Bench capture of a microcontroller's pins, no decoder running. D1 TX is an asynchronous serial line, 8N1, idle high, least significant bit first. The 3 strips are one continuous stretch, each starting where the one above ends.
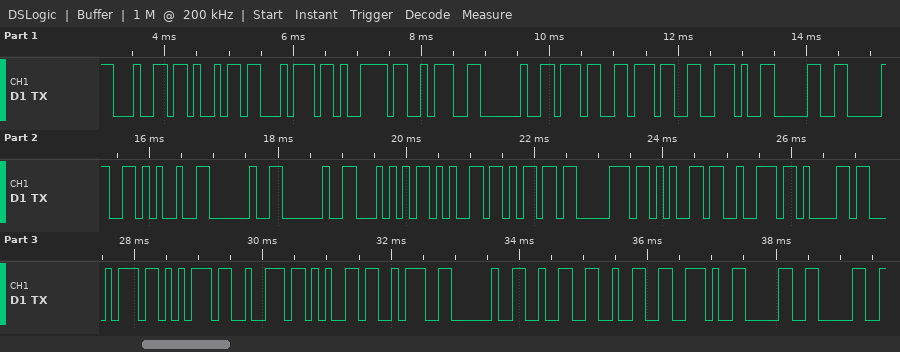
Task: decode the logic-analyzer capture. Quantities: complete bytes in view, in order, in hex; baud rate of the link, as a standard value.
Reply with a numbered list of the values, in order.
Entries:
1. 64 69 74 79 3A 20 37 37 2E 30 30 25 20 20 54 65 6D 70 65 72 61 74 75 72 65 3A 20 32 32 2E 30 30
2. 9600 baud
